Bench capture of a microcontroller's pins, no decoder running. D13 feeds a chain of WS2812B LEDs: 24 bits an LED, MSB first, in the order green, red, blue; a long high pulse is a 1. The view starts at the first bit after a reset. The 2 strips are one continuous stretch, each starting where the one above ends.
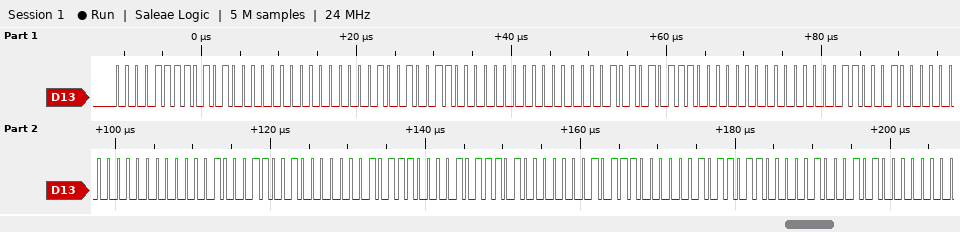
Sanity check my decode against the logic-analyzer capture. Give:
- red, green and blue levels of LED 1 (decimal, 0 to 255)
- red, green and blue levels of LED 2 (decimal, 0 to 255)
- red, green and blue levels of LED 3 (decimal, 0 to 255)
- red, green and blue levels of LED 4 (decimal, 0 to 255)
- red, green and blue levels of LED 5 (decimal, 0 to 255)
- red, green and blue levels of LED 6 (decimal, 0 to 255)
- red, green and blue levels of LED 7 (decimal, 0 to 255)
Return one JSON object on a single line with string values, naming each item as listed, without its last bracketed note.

{"red, green and blue levels of LED 1": "80, 15, 0", "red, green and blue levels of LED 2": "96, 18, 0", "red, green and blue levels of LED 3": "112, 21, 0", "red, green and blue levels of LED 4": "128, 24, 0", "red, green and blue levels of LED 5": "144, 17, 23", "red, green and blue levels of LED 6": "160, 11, 46", "red, green and blue levels of LED 7": "176, 5, 69"}
